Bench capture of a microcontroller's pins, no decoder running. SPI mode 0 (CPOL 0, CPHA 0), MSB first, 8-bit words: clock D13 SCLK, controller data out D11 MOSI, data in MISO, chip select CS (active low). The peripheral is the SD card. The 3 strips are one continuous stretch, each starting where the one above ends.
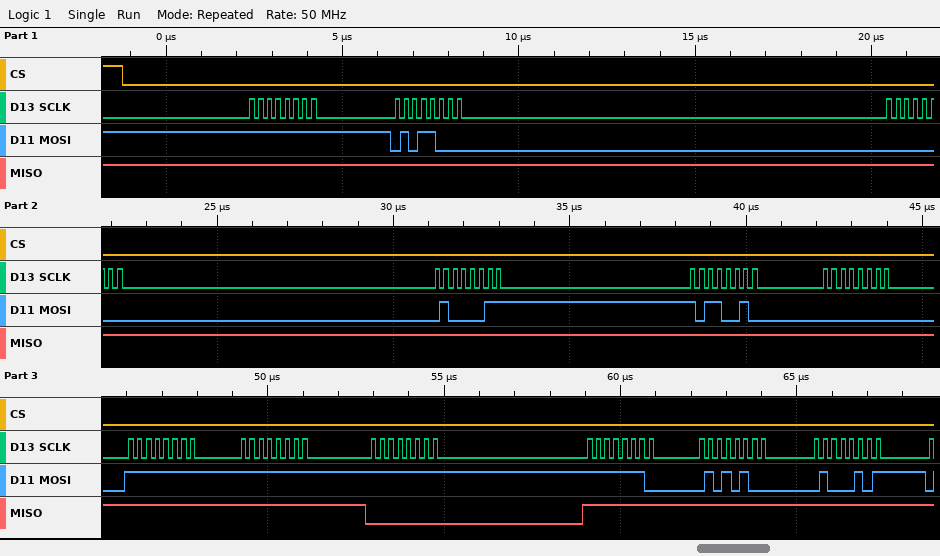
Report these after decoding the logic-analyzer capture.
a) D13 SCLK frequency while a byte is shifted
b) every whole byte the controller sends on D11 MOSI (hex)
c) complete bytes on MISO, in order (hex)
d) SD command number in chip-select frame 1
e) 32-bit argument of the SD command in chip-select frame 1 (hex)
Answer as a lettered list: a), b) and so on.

a) 4 MHz
b) FF 58 00 43 B2 00 FF FF FF FE 54 45
c) FF FF FF FF FF FF FF FF 00 FF FF FF
d) CMD24
e) 0x0043B200
